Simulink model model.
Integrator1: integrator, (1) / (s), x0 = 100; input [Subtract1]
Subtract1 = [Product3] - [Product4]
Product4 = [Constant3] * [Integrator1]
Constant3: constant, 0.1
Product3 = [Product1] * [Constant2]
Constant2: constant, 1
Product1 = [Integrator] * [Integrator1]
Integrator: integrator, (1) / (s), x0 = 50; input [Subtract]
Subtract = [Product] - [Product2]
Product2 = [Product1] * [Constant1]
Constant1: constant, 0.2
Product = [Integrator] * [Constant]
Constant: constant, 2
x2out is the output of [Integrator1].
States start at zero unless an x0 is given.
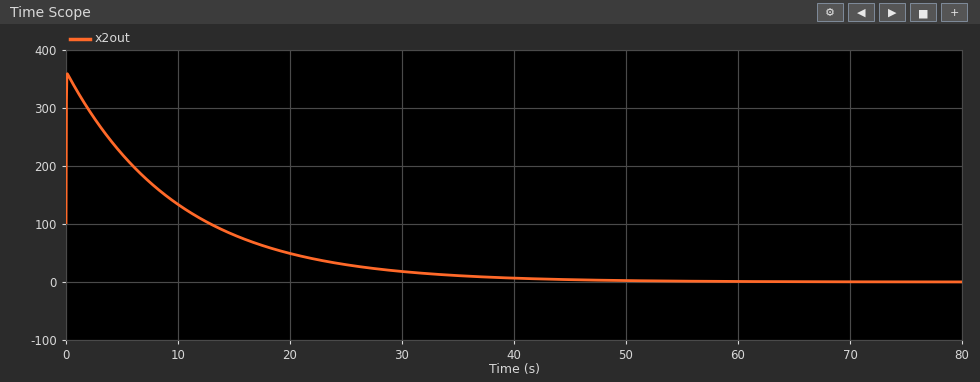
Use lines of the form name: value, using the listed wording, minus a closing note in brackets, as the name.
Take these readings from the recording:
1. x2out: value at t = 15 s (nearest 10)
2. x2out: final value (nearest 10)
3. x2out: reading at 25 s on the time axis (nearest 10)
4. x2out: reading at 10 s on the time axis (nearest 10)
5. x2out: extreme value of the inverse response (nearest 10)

x2out: value at t = 15 s: 80
x2out: final value: 0
x2out: reading at 25 s on the time axis: 30
x2out: reading at 10 s on the time axis: 130
x2out: extreme value of the inverse response: 360
